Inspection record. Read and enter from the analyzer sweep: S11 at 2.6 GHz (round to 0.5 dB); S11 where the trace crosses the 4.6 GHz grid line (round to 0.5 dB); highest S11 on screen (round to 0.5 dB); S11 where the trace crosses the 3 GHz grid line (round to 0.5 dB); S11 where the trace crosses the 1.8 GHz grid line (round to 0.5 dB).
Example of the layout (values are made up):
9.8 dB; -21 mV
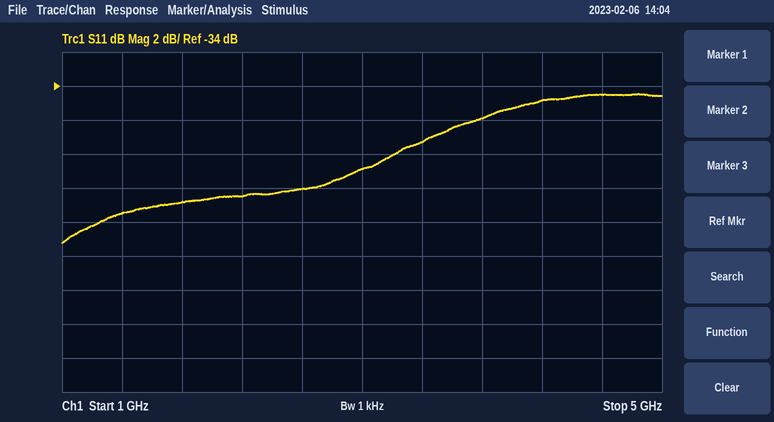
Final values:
-40.0 dB; -34.5 dB; -34.5 dB; -39.0 dB; -41.0 dB
